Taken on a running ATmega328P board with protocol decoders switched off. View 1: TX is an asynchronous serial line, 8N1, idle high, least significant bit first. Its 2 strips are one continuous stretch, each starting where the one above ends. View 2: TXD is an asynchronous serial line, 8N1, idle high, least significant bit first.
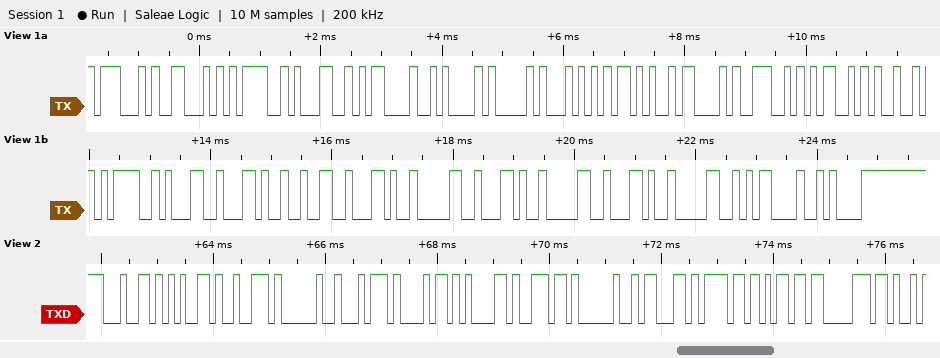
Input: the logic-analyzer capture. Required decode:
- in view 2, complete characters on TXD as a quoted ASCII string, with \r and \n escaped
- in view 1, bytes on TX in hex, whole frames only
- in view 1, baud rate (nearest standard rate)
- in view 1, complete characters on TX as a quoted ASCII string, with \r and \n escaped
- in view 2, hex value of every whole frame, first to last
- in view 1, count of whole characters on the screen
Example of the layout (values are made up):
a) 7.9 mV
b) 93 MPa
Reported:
a) "der than comp"
b) 47 46 3D 31 0D 0A 41 54 2B 43 4E 4D 49 3D 31 2C 32 2C 30 2C 30 2C 30 0D 0A
c) 9600 baud
d) "GF=1\r\nAT+CNMI=1,2,0,0,0\r\n"
e) 0x64 0x65 0x72 0x20 0x74 0x68 0x61 0x6E 0x20 0x63 0x6F 0x6D 0x70
f) 25
